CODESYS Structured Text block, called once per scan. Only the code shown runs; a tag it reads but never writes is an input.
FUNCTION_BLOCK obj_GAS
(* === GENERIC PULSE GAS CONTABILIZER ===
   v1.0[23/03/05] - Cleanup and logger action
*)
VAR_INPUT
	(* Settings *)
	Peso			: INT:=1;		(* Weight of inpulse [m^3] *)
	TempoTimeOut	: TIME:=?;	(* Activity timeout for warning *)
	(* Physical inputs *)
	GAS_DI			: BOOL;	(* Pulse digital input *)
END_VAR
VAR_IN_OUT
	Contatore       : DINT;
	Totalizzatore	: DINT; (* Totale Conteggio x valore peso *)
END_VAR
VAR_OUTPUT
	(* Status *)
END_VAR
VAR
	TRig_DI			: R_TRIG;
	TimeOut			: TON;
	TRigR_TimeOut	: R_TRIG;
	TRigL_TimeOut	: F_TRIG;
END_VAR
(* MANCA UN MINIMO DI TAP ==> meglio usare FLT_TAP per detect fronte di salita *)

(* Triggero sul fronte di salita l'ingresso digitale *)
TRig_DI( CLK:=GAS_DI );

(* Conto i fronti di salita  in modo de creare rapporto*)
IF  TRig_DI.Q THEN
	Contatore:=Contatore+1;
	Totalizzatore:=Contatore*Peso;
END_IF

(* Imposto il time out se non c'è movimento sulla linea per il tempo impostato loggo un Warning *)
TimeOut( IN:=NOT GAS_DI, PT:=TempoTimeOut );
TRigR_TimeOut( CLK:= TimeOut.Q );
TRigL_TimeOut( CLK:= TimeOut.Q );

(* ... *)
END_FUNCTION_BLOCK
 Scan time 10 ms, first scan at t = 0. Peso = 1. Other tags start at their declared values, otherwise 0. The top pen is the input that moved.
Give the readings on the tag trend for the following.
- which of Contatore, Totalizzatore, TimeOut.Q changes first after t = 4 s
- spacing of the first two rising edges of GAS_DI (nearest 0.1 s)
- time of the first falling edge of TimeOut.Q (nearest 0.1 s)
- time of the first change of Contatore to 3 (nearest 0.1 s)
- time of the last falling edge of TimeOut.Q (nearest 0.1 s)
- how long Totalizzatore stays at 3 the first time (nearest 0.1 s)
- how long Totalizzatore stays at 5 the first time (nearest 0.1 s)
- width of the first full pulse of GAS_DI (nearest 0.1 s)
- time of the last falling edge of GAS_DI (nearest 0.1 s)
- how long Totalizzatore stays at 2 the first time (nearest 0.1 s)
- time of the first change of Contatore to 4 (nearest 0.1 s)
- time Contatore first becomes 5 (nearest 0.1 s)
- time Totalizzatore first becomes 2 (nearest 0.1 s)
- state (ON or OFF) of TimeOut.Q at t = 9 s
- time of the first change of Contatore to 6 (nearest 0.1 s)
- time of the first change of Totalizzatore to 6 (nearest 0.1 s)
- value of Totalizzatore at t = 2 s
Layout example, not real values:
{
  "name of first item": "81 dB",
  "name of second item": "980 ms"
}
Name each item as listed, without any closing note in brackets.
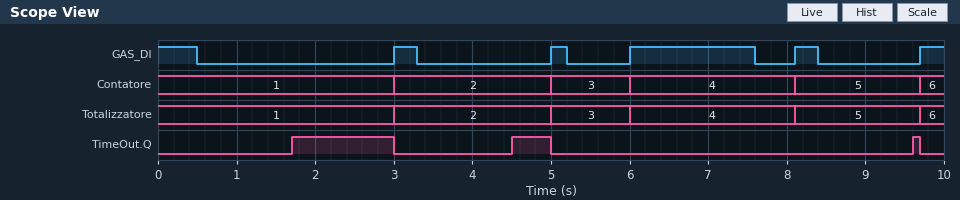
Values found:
{
  "which of Contatore, Totalizzatore, TimeOut.Q changes first after t = 4 s": "TimeOut.Q",
  "spacing of the first two rising edges of GAS_DI": "2.0 s",
  "time of the first falling edge of TimeOut.Q": "3.0 s",
  "time of the first change of Contatore to 3": "5.0 s",
  "time of the last falling edge of TimeOut.Q": "9.7 s",
  "how long Totalizzatore stays at 3 the first time": "1.0 s",
  "how long Totalizzatore stays at 5 the first time": "1.6 s",
  "width of the first full pulse of GAS_DI": "0.3 s",
  "time of the last falling edge of GAS_DI": "8.4 s",
  "how long Totalizzatore stays at 2 the first time": "2.0 s",
  "time of the first change of Contatore to 4": "6.0 s",
  "time Contatore first becomes 5": "8.1 s",
  "time Totalizzatore first becomes 2": "3.0 s",
  "state (ON or OFF) of TimeOut.Q at t = 9 s": "OFF",
  "time of the first change of Contatore to 6": "9.7 s",
  "time of the first change of Totalizzatore to 6": "9.7 s",
  "value of Totalizzatore at t = 2 s": "1"
}
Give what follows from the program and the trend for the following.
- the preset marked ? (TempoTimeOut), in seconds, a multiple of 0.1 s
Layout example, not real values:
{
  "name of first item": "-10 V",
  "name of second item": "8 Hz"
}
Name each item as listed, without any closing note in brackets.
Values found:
{
  "the preset marked ? (TempoTimeOut), in seconds, a multiple of 0.1 s": "1.2 s"
}
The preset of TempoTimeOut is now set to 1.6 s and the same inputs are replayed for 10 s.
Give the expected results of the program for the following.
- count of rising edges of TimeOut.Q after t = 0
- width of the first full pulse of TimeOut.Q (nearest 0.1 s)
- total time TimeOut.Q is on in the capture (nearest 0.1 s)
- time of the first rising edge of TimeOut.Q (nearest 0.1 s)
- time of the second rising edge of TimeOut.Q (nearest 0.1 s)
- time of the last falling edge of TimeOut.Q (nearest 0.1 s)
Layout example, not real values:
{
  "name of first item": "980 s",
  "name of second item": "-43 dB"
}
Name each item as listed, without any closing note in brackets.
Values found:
{
  "count of rising edges of TimeOut.Q after t = 0": "2",
  "width of the first full pulse of TimeOut.Q": "0.9 s",
  "total time TimeOut.Q is on in the capture": "1.0 s",
  "time of the first rising edge of TimeOut.Q": "2.1 s",
  "time of the second rising edge of TimeOut.Q": "4.9 s",
  "time of the last falling edge of TimeOut.Q": "5.0 s"
}
